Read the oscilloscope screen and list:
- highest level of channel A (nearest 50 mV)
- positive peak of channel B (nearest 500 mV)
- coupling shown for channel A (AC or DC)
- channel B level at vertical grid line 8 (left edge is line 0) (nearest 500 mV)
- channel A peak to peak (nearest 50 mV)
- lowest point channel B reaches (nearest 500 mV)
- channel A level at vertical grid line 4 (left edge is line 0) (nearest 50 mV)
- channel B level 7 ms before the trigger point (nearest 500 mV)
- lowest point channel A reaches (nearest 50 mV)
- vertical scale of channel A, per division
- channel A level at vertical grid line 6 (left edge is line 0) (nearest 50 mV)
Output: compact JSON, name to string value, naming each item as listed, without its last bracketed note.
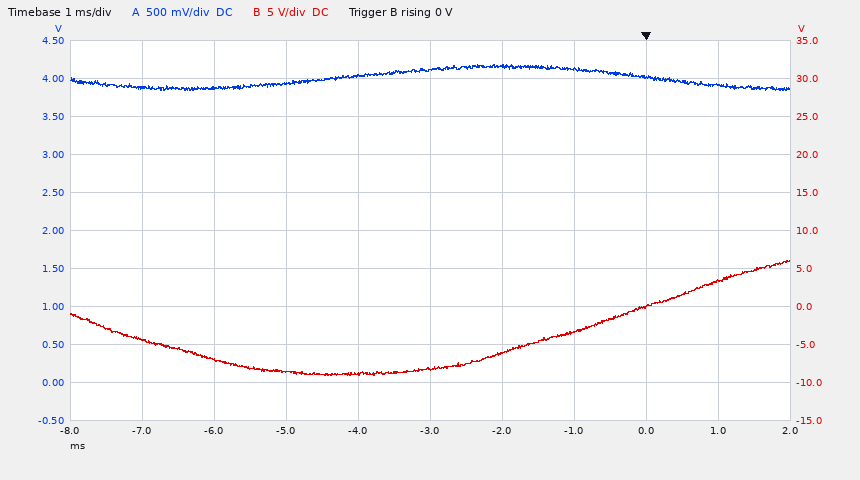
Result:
{"highest level of channel A": "4.20 V", "positive peak of channel B": "6.0 V", "coupling shown for channel A": "DC", "channel B level at vertical grid line 8 (left edge is line 0)": "0.0 V", "channel A peak to peak": "350 mV", "lowest point channel B reaches": "-9.0 V", "channel A level at vertical grid line 4 (left edge is line 0)": "4.05 V", "channel B level 7 ms before the trigger point": "-4.5 V", "lowest point channel A reaches": "3.85 V", "vertical scale of channel A, per division": "500 mV", "channel A level at vertical grid line 6 (left edge is line 0)": "4.15 V"}
